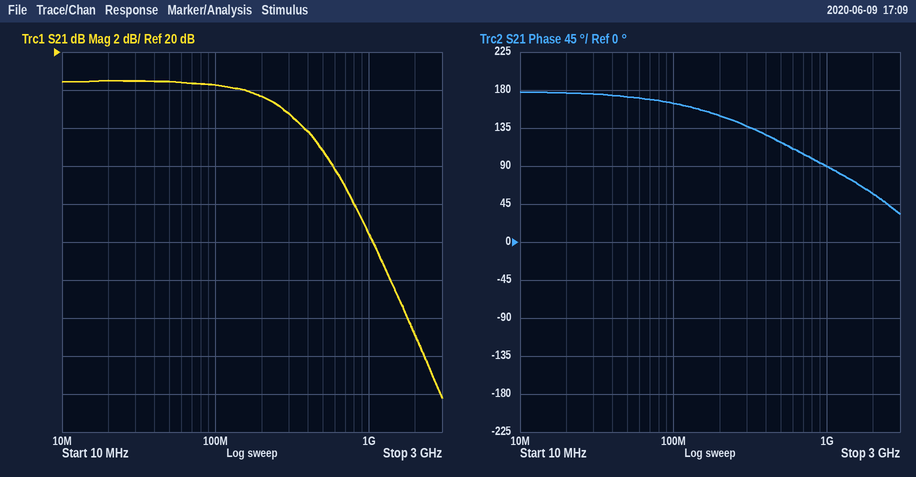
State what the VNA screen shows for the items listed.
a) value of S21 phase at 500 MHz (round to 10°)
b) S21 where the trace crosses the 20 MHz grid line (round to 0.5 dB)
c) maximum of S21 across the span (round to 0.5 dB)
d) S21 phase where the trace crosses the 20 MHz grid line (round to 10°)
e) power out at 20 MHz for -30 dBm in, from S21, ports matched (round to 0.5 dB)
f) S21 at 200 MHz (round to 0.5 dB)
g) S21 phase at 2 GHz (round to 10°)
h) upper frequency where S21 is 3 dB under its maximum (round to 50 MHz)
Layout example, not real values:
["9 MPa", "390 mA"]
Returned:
["120°", "18.5 dB", "18.5 dB", "180°", "-11.5 dBm", "17.5 dB", "60°", "450 MHz"]
